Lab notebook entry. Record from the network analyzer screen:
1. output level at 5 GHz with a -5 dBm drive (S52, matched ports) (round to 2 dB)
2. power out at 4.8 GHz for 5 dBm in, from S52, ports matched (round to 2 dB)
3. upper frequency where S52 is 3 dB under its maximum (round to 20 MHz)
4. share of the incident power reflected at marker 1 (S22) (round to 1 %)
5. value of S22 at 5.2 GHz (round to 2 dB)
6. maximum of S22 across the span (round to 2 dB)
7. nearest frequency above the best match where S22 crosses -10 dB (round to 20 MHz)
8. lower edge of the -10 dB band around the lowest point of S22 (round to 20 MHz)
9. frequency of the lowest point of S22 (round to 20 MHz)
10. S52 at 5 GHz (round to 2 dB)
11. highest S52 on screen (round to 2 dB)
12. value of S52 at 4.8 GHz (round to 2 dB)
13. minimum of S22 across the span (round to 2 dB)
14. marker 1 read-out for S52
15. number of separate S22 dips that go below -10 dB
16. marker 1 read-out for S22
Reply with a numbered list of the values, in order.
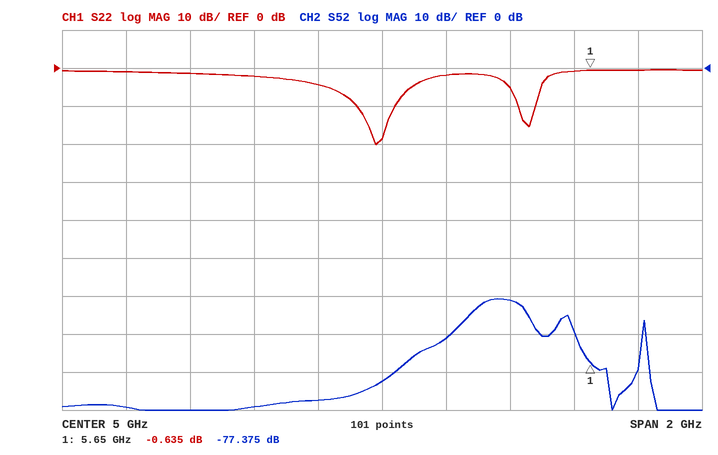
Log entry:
1. -88 dBm
2. -82 dBm
3. 5.44 GHz
4. 86 %
5. -2 dB
6. 0 dB
7. 5.04 GHz
8. 4.92 GHz
9. 4.98 GHz
10. -82 dB
11. -60 dB
12. -88 dB
13. -20 dB
14. -77.375 dB
15. 2
16. -0.635 dB
